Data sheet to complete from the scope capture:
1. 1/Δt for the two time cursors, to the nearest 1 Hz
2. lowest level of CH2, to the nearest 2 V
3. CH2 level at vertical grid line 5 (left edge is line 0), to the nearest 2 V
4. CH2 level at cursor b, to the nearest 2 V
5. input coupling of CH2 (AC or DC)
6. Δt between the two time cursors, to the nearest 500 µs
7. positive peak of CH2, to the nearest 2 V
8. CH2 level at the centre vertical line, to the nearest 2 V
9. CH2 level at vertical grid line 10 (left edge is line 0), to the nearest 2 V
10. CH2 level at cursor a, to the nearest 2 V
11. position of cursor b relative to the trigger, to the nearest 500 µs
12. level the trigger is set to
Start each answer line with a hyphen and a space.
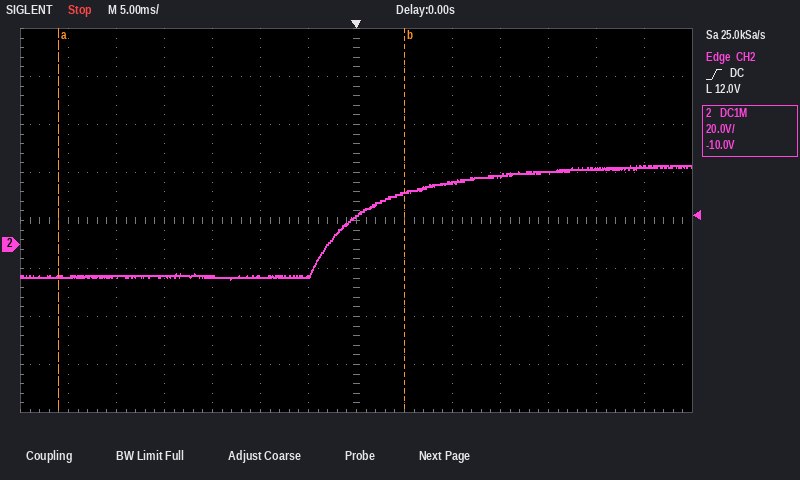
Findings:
- 28 Hz
- -14 V
- -14 V
- 22 V
- DC
- 36.0 ms
- 32 V
- 12 V
- 28 V
- -14 V
- +5.0 ms
- 12.0 V
